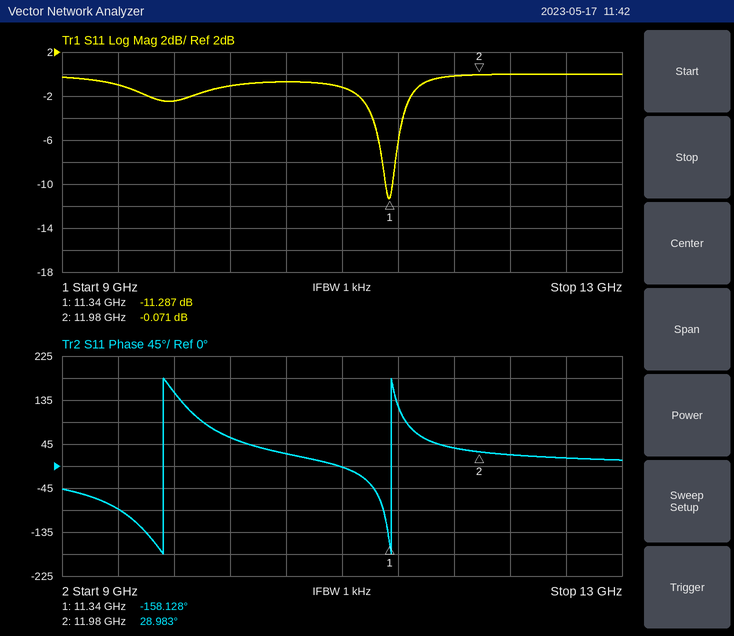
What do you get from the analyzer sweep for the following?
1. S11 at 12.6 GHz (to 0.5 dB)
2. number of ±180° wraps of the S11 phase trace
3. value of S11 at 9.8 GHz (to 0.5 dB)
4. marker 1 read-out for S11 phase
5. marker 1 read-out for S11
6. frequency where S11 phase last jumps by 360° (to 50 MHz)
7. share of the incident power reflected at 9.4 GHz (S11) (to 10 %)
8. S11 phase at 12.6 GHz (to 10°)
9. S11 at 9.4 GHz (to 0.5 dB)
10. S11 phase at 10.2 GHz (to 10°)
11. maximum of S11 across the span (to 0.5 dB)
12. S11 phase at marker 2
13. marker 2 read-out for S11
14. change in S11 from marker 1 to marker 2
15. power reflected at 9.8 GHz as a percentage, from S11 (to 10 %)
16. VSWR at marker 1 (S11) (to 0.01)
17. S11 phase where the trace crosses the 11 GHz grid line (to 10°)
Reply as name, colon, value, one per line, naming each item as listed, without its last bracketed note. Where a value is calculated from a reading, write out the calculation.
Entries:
S11 at 12.6 GHz: 0.0 dB
number of ±180° wraps of the S11 phase trace: 2
value of S11 at 9.8 GHz: -2.5 dB
marker 1 read-out for S11 phase: -158.128°
marker 1 read-out for S11: -11.287 dB
frequency where S11 phase last jumps by 360°: 11.35 GHz
share of the incident power reflected at 9.4 GHz (S11): 10^(-1/10) ≈ 79.4 %, so 80 % to the nearest 10 %
S11 phase at 12.6 GHz: 20°
S11 at 9.4 GHz: -1.0 dB
S11 phase at 10.2 GHz: 60°
maximum of S11 across the span: 0.0 dB
S11 phase at marker 2: 28.983°
marker 2 read-out for S11: -0.071 dB
change in S11 from marker 1 to marker 2: -0.071 − (-11.287) = 11.216 dB
power reflected at 9.8 GHz as a percentage, from S11: 10^(-2.5/10) ≈ 56.2 %, so 60 % to the nearest 10 %
VSWR at marker 1 (S11): (1 + 0.2727)/(1 − 0.2727) ≈ 1.75
S11 phase where the trace crosses the 11 GHz grid line: 0°
